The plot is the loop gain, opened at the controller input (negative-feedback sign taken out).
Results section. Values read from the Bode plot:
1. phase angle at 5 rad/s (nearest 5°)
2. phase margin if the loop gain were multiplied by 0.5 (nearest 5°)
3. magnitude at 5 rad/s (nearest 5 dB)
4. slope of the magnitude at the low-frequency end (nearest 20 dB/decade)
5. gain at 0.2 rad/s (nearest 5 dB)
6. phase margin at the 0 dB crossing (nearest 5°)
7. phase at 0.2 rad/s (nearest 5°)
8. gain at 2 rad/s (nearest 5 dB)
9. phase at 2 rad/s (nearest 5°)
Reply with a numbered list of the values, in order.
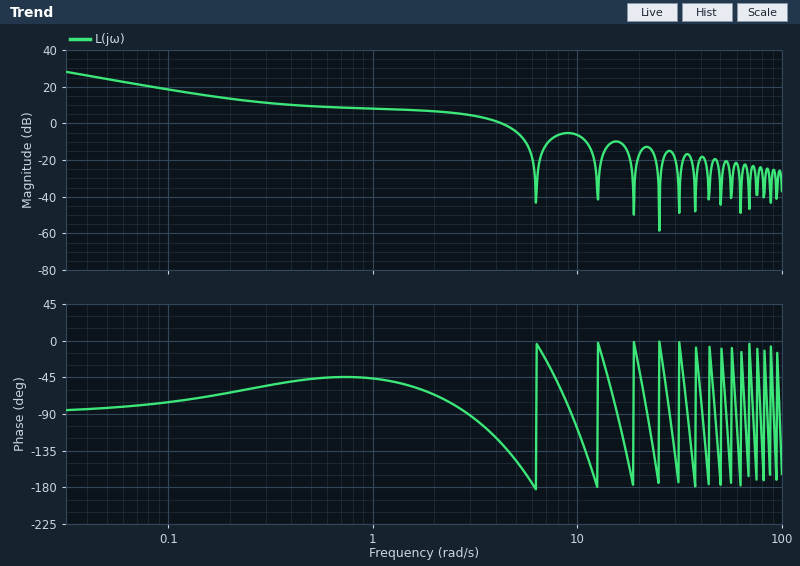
1. -145°
2. 105°
3. -5 dB
4. -20 dB/decade
5. 15 dB
6. 55°
7. -65°
8. 5 dB
9. -65°
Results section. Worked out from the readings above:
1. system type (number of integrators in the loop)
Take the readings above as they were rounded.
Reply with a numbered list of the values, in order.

1. 1
